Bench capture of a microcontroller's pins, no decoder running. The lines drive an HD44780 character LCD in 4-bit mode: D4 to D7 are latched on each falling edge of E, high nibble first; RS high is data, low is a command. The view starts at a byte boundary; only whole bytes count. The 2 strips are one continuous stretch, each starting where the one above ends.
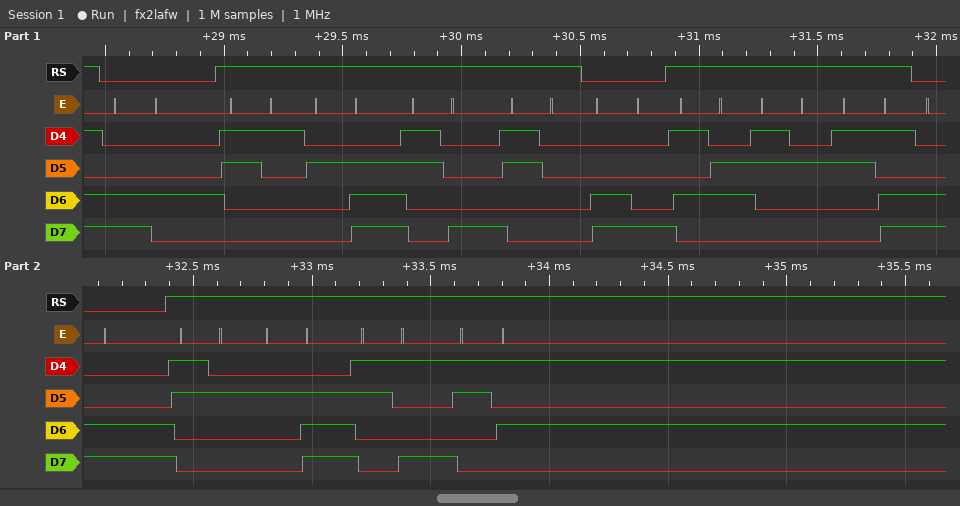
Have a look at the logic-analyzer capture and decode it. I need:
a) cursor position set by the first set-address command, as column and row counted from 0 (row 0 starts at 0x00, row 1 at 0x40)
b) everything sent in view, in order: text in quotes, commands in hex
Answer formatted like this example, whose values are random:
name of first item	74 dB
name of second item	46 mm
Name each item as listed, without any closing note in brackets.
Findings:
cursor position set by the first set-address command, as column and row counted from 0	column 4, row 1
everything sent in view, in order: text in quotes, commands in hex	0xC4 "1.80" 0xC8 "V2=" 0xCC "2.95"
